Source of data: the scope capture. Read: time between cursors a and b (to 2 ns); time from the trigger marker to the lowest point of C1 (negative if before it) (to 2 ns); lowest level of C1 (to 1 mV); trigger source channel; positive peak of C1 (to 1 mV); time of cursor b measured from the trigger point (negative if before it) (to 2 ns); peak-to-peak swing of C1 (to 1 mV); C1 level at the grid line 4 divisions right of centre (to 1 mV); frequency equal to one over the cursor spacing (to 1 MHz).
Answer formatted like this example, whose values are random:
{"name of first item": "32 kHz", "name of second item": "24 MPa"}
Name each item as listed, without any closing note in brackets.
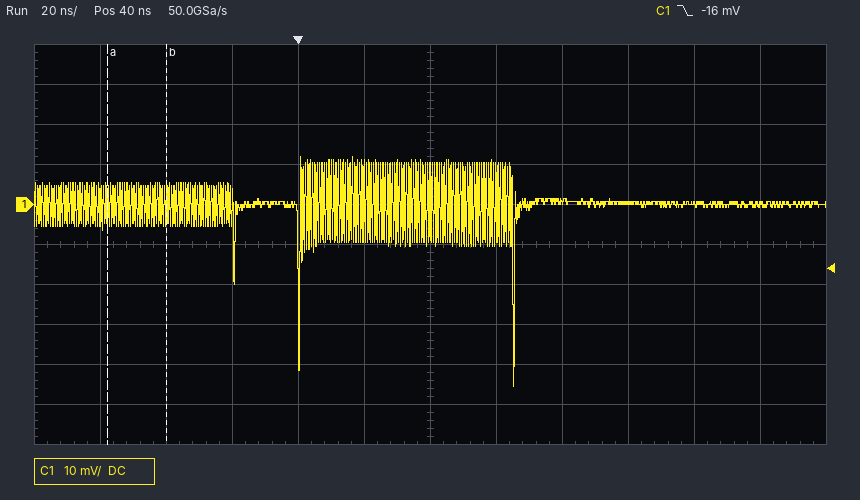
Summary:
{"time between cursors a and b": "18 ns", "time from the trigger marker to the lowest point of C1 (negative if before it)": "+66 ns", "lowest level of C1": "-46 mV", "trigger source channel": "C1", "positive peak of C1": "12 mV", "time of cursor b measured from the trigger point (negative if before it)": "-40 ns", "peak-to-peak swing of C1": "58 mV", "C1 level at the grid line 4 divisions right of centre": "0 mV", "frequency equal to one over the cursor spacing": "56 MHz"}
